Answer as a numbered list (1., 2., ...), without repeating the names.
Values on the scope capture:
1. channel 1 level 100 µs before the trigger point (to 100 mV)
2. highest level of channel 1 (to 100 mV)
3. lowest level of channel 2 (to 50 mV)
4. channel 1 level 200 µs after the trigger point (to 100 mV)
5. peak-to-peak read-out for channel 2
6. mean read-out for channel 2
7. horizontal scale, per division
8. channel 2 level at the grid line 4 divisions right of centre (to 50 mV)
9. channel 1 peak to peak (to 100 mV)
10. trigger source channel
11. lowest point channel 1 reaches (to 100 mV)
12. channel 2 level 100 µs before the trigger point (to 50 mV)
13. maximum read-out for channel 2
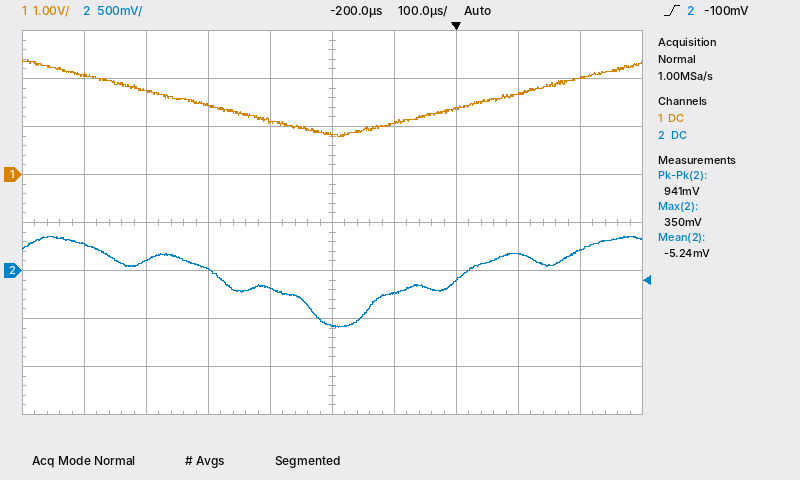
1. 1.1 V
2. 2.4 V
3. -600 mV
4. 2.0 V
5. 941 mV
6. -5.24 mV
7. 100 µs
8. 200 mV
9. 1.6 V
10. channel 2
11. 800 mV
12. -250 mV
13. 350 mV
